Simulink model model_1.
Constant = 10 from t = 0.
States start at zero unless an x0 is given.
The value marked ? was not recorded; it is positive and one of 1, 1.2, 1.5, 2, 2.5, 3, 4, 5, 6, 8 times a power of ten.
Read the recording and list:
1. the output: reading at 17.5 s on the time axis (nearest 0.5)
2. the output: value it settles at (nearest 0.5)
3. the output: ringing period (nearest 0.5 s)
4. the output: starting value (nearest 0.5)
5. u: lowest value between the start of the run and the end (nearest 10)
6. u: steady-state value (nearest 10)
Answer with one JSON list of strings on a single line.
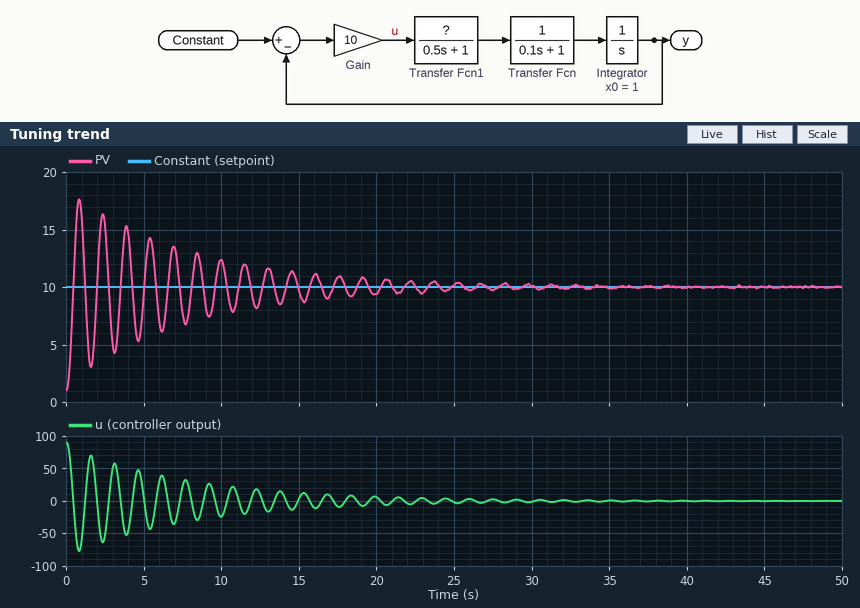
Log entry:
["11.0", "10.0", "1.5 s", "1.0", "-80", "0"]
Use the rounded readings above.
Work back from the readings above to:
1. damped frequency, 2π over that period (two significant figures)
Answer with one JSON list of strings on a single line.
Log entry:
["4.2 rad/s"]
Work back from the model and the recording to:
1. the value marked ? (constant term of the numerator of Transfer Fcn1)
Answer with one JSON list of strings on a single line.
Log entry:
["1"]
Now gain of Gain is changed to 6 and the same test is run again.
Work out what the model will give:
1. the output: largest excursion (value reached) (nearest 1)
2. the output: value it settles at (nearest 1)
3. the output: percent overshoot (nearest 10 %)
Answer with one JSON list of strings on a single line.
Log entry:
["16", "10", "60 %"]
